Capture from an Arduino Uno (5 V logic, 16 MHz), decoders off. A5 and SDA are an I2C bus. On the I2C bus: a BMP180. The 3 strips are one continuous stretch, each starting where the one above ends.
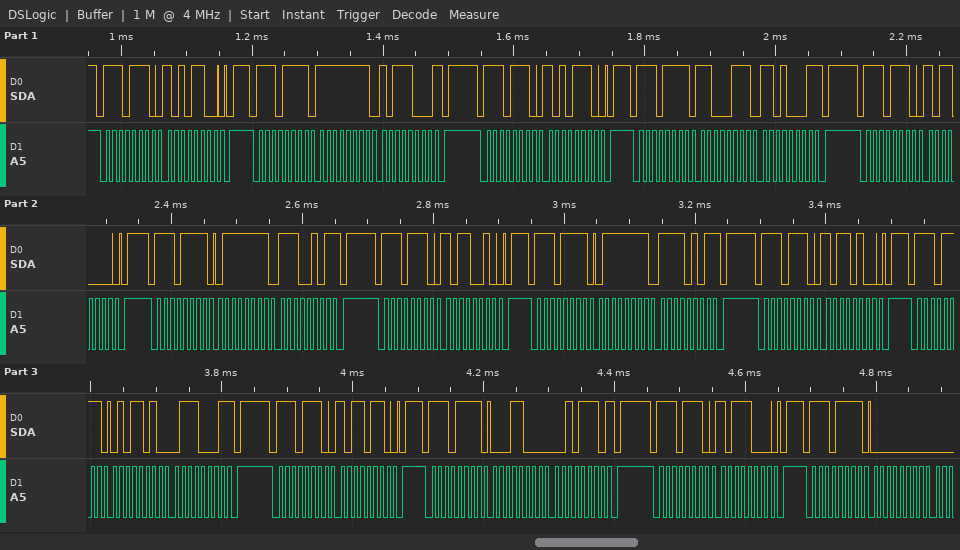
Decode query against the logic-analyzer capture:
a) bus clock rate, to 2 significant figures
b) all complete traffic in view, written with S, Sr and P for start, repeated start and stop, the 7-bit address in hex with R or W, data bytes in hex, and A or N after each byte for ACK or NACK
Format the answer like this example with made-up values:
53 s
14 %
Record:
100 kHz
S 77W A AC A P S 77R A FF A B8 N P S 77W A AE A P S 77R A C7 A D1 N P S 77W A B0 A P S 77R A 7F A E5 N P S 77W A B2 A P S 77R A 7F A F5 N P S 77W A B4 A P S 77R A 5A A 71 N P S 77W A B6 A P S 77R A 18 A 2E N P S 77W A B8 A P S 77R A 00 A
